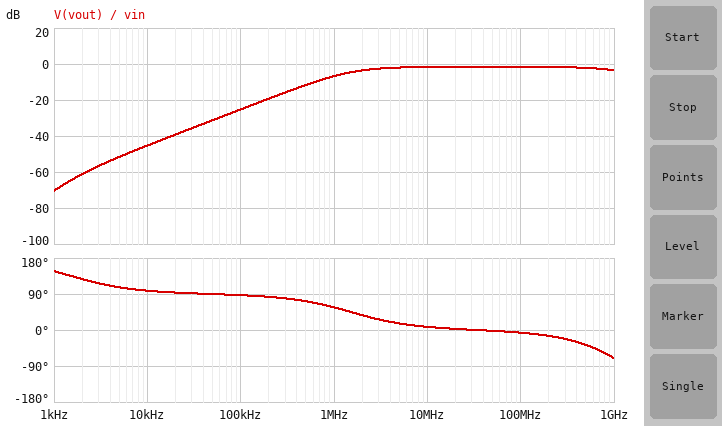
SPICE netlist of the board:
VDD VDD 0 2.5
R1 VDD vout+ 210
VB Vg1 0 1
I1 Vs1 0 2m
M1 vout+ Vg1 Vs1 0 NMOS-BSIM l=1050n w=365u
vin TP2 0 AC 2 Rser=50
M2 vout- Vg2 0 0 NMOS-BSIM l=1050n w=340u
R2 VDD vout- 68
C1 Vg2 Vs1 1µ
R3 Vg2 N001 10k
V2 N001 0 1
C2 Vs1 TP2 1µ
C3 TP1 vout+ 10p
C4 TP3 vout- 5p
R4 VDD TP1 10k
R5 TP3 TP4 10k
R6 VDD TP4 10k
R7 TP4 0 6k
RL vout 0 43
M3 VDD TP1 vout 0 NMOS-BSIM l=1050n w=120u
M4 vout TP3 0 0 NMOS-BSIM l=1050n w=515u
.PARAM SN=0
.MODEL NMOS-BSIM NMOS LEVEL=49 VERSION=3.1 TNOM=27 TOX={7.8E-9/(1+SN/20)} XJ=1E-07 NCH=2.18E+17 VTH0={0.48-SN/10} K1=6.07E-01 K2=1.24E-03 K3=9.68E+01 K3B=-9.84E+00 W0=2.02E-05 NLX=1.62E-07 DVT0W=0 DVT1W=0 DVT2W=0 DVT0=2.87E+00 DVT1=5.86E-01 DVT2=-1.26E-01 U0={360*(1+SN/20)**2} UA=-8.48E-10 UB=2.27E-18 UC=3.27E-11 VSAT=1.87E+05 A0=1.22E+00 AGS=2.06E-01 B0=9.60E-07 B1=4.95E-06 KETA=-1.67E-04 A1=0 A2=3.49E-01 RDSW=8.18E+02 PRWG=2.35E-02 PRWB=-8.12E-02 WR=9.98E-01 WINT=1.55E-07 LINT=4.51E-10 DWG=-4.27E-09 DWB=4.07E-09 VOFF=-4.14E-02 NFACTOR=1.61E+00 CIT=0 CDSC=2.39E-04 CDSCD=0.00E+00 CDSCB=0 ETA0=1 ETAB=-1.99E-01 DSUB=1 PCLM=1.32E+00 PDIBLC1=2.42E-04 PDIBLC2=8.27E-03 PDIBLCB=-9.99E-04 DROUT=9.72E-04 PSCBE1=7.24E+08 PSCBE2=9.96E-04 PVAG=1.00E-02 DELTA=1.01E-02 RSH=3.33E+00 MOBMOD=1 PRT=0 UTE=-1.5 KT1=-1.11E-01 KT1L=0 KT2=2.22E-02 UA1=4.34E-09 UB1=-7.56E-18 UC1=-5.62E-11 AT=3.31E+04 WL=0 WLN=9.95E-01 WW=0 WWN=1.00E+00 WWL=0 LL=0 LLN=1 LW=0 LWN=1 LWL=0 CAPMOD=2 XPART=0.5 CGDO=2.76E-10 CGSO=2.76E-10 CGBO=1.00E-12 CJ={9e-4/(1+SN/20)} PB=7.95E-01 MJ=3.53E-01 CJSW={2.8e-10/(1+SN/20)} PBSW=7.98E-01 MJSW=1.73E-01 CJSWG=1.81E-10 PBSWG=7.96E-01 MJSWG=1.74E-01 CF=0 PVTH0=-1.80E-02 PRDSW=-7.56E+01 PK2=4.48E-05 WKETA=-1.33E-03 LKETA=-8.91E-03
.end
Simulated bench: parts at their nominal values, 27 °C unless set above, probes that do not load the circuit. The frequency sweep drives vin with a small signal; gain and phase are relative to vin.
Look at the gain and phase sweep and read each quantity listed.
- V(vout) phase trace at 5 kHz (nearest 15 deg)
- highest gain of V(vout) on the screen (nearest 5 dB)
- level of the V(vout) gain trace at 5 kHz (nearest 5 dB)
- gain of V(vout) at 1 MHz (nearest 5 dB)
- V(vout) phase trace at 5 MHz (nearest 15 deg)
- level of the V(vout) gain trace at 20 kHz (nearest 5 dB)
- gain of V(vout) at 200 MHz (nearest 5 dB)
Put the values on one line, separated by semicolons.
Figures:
105 deg; 0 dB; -50 dB; -5 dB; 15 deg; -40 dB; 0 dB
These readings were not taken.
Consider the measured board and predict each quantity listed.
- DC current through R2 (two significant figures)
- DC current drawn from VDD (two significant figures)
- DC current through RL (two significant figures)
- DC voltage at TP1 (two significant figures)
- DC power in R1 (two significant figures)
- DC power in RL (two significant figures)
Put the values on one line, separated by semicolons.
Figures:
4.9 mA; 21 mA; 8.5 mA; 2.5 V; 840 µW; 3.1 mW
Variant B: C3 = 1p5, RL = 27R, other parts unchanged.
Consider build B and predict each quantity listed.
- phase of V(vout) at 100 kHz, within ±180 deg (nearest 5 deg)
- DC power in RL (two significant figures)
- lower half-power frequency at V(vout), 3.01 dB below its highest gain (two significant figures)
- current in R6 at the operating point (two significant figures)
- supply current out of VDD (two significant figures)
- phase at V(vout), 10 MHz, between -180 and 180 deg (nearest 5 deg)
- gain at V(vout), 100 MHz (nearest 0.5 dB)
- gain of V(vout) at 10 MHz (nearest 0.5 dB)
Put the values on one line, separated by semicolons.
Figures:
90 deg; 2.9 mW; 7.2 MHz; 160 µA; 22 mA; 30 deg; -6.0 dB; -8.0 dB
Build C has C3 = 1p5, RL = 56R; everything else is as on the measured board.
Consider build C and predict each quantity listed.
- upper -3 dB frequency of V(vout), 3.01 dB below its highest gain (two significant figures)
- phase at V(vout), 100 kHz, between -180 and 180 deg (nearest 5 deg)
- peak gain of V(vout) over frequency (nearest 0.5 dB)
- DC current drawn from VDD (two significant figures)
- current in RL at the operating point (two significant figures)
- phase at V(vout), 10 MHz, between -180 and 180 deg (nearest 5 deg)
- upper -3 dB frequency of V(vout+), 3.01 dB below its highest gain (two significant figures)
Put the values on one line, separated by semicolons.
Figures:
1.4 GHz; 90 deg; -1.0 dB; 20 mA; 7.5 mA; 30 deg; 1.6 GHz
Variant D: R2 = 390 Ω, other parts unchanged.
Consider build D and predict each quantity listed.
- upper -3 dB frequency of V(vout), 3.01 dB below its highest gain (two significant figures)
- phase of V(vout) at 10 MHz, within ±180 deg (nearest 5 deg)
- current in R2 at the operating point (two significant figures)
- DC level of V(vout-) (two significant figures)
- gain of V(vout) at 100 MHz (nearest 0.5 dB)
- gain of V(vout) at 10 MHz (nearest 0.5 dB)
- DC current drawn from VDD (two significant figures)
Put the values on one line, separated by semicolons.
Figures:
320 MHz; 5 deg; 4.7 mA; 680 mV; 4.0 dB; 4.5 dB; 20 mA
